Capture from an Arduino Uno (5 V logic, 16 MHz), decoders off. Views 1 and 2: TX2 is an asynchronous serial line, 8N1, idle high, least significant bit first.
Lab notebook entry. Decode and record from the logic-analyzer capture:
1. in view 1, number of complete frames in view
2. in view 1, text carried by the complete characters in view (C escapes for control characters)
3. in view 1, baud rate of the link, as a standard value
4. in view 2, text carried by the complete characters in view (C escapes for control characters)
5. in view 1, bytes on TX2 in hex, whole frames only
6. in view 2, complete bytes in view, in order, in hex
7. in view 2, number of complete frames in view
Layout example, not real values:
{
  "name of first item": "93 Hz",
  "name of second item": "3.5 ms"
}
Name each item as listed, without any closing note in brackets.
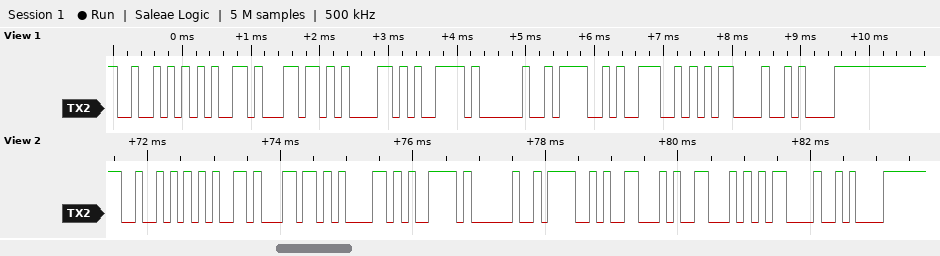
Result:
{
  "in view 1, number of complete frames in view": "10",
  "in view 1, text carried by the complete characters in view": "\"Relay ON\\r\\n\"",
  "in view 1, baud rate of the link, as a standard value": "9600 baud",
  "in view 2, text carried by the complete characters in view": "\"Relay OFF\\r\\n\"",
  "in view 1, bytes on TX2 in hex, whole frames only": "0x52 0x65 0x6C 0x61 0x79 0x20 0x4F 0x4E 0x0D 0x0A",
  "in view 2, complete bytes in view, in order, in hex": "52 65 6C 61 79 20 4F 46 46 0D 0A",
  "in view 2, number of complete frames in view": "11"
}
